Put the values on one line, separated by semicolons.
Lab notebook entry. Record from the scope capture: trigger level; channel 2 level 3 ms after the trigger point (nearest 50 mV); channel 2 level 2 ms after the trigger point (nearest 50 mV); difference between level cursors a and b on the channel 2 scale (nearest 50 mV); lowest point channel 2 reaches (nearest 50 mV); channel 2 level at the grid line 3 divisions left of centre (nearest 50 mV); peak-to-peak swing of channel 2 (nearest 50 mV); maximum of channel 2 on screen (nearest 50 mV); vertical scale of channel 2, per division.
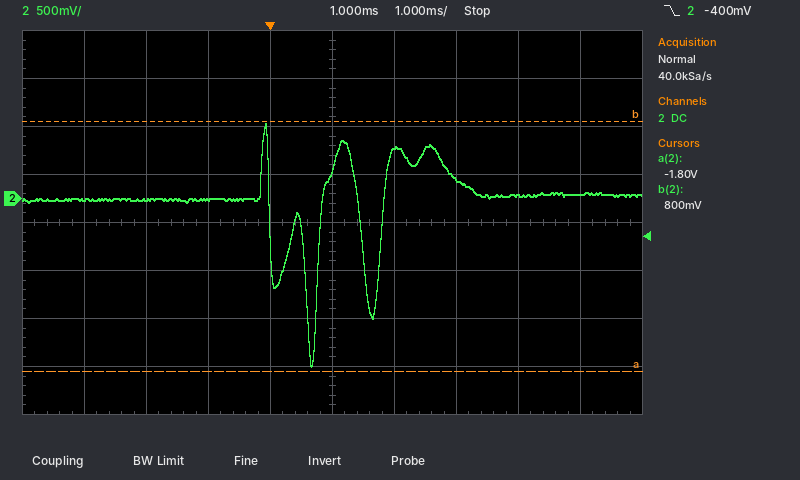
-400 mV; 200 mV; 500 mV; 2.60 V; -1.75 V; 0 mV; 2.55 V; 800 mV; 500 mV
